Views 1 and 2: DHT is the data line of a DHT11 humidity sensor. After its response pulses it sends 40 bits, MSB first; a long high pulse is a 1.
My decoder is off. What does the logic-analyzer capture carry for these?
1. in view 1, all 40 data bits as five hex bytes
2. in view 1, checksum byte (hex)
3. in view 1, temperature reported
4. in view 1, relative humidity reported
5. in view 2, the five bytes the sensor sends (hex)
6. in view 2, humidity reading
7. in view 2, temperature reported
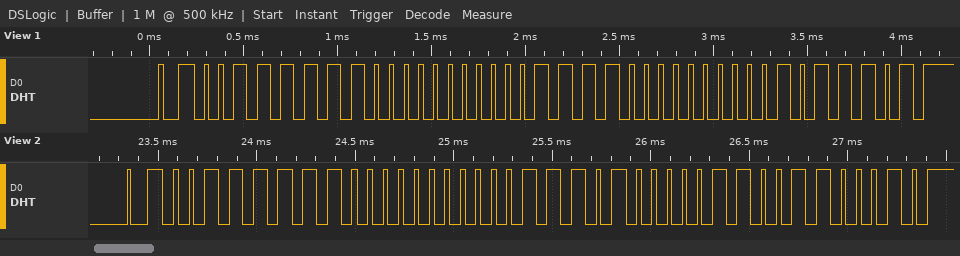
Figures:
3F 00 1E 00 5D
0x5D
30.0 °C
63 %
3F 00 1D 06 62
63 %
29.6 °C
